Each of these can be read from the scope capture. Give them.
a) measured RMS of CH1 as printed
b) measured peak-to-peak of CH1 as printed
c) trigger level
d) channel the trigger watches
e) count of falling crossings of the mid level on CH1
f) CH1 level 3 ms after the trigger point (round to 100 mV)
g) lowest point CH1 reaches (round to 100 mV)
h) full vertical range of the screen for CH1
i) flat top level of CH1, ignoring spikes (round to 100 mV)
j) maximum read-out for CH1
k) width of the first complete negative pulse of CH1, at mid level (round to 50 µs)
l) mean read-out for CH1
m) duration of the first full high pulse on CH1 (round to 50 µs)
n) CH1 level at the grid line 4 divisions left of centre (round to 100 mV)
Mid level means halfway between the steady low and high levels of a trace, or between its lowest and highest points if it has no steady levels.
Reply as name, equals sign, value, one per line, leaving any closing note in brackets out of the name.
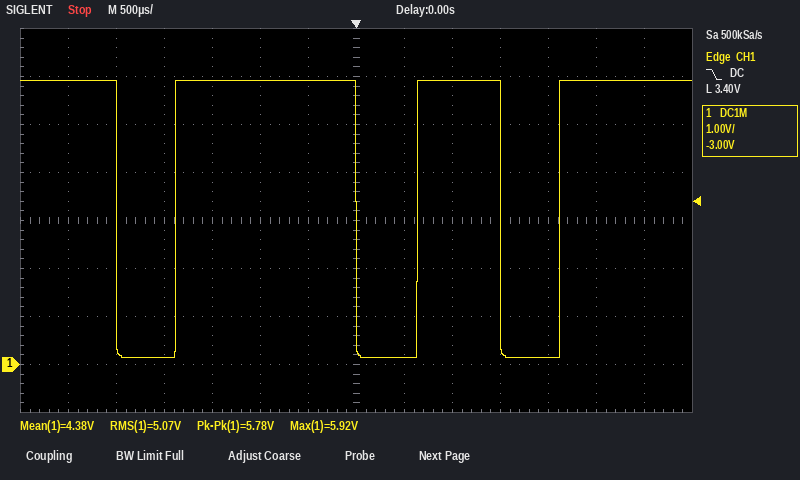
measured RMS of CH1 as printed = 5.07 V
measured peak-to-peak of CH1 as printed = 5.78 V
trigger level = 3.40 V
channel the trigger watches = CH1
count of falling crossings of the mid level on CH1 = 3
CH1 level 3 ms after the trigger point = 5.9 V
lowest point CH1 reaches = 100 mV
full vertical range of the screen for CH1 = 8 V
flat top level of CH1, ignoring spikes = 5.9 V
maximum read-out for CH1 = 5.92 V
width of the first complete negative pulse of CH1, at mid level = 600 µs
mean read-out for CH1 = 4.38 V
duration of the first full high pulse on CH1 = 1.90 ms
CH1 level at the grid line 4 divisions left of centre = 100 mV
